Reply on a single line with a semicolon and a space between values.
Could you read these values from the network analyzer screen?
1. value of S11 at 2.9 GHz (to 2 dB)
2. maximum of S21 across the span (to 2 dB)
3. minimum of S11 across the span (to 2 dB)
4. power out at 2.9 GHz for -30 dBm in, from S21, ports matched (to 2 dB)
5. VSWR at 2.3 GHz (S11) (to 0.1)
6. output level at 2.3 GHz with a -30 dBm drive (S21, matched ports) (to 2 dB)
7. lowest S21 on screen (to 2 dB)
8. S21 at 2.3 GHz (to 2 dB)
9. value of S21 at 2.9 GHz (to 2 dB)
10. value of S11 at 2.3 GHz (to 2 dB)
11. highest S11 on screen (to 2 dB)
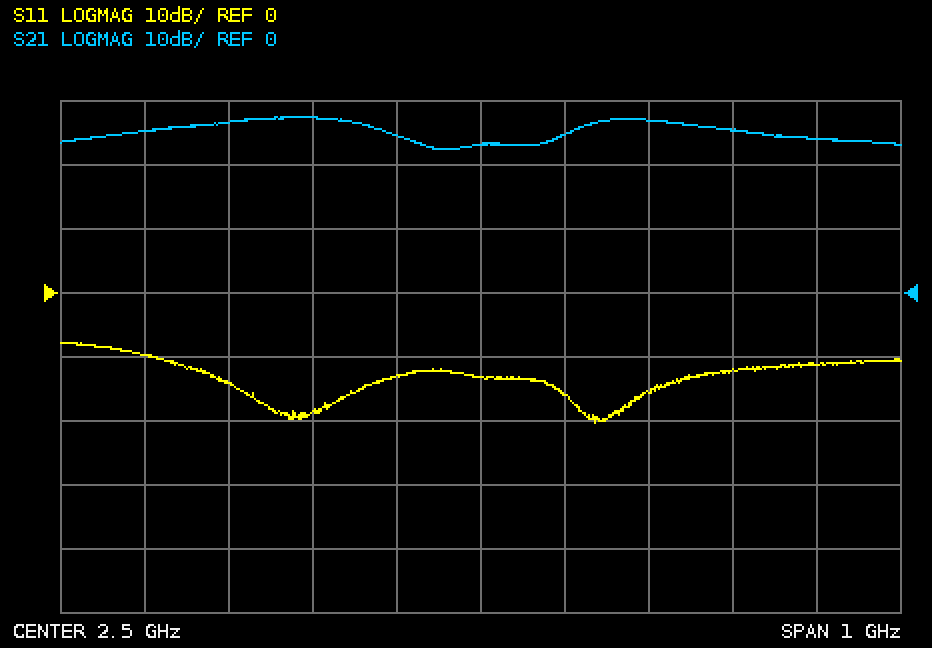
-12 dB; 28 dB; -20 dB; -6 dBm; 1.3; -2 dBm; 22 dB; 28 dB; 24 dB; -18 dB; -8 dB
